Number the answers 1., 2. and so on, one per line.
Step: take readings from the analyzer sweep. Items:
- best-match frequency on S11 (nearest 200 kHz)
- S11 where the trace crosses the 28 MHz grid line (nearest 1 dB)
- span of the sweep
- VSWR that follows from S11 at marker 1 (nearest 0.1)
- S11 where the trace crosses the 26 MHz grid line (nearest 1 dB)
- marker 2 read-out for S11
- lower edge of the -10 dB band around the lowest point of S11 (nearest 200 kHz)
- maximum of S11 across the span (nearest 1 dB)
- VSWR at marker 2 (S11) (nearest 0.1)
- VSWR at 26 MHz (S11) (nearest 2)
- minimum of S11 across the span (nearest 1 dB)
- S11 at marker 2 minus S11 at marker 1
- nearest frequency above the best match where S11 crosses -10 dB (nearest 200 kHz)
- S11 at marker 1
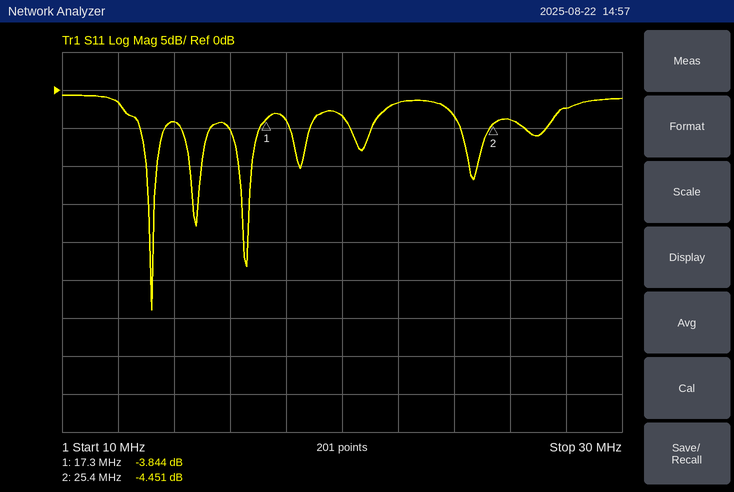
1. 13.2 MHz
2. -2 dB
3. 20 MHz
4. 4.6
5. -4 dB
6. -4.451 dB
7. 13.0 MHz
8. -1 dB
9. 4.0
10. 4
11. -29 dB
12. -0.607 dB
13. 13.4 MHz
14. -3.844 dB
